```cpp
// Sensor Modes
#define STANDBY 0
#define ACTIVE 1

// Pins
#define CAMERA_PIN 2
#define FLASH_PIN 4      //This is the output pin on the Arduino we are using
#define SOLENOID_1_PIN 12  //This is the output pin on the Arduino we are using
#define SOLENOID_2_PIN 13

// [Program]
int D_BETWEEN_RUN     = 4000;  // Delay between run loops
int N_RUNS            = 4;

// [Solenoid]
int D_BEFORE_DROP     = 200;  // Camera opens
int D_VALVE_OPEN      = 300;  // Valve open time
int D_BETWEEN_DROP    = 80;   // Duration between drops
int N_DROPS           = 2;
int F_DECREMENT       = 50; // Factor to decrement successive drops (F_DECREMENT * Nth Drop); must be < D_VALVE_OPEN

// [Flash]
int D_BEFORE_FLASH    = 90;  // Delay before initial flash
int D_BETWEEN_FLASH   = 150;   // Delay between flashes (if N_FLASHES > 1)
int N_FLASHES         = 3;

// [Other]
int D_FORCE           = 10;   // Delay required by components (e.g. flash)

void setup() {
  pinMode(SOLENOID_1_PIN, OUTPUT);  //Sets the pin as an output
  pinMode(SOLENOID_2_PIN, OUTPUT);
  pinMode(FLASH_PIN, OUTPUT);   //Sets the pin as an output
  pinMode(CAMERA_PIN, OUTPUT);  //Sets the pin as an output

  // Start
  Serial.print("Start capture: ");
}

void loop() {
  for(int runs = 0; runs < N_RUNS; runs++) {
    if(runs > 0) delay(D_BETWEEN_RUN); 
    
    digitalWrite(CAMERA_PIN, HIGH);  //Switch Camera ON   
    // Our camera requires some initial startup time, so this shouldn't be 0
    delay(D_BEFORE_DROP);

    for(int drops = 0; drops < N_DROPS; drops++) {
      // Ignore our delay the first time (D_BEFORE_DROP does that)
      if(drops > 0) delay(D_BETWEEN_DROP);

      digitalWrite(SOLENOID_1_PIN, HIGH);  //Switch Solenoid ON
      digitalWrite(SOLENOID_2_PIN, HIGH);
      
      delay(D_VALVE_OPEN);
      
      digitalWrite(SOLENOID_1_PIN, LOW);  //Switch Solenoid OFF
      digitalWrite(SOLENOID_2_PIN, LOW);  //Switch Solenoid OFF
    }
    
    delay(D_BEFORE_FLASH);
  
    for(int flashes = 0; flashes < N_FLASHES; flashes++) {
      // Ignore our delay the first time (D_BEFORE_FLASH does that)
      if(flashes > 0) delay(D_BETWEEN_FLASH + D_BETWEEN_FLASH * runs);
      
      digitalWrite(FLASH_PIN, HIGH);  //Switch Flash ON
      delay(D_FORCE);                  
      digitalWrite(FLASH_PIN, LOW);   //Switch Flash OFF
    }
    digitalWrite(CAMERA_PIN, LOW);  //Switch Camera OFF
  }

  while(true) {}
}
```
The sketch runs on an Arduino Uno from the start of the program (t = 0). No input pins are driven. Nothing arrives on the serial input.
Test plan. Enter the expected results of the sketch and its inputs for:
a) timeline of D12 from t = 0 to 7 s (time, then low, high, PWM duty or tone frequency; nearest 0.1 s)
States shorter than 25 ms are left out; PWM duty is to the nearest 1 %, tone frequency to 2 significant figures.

0 s low; 0.2 s high; 0.5 s low; 0.6 s high; 0.9 s low; 5.5 s high; 5.8 s low; 5.9 s high; 6.2 s low
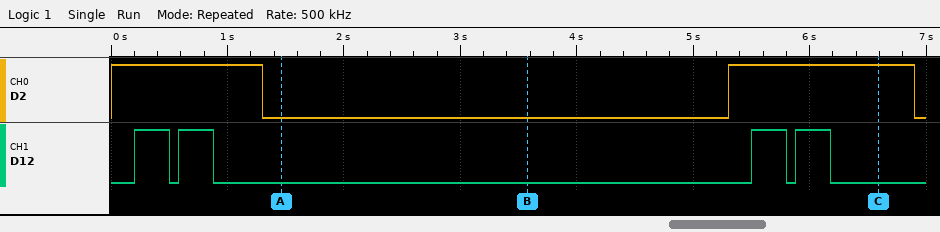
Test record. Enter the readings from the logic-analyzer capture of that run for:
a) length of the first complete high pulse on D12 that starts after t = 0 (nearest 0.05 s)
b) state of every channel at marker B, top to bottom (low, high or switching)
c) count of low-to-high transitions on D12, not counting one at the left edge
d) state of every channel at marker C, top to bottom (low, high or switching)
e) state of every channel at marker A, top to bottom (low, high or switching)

0.30 s
D2 low, D12 low
4
D2 high, D12 low
D2 low, D12 low
